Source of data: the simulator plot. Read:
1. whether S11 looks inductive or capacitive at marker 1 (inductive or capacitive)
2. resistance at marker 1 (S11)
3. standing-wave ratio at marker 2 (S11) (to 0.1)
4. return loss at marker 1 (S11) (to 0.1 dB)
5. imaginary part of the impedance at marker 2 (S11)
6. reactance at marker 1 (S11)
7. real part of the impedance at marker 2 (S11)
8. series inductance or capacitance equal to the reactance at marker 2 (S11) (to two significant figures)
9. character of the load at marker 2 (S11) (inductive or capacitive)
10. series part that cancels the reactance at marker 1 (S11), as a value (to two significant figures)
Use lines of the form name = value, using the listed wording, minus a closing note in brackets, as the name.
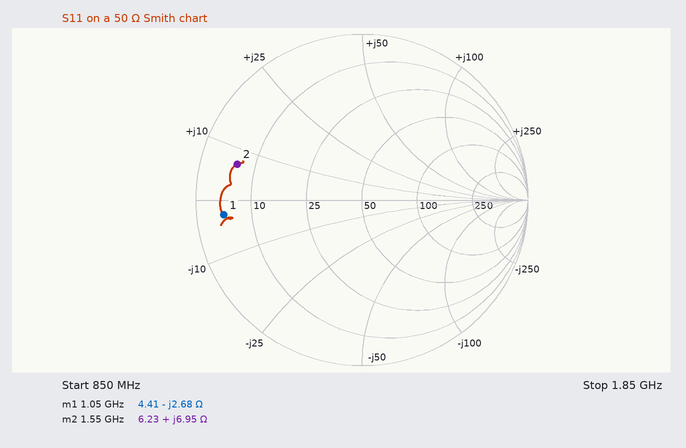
whether S11 looks inductive or capacitive at marker 1 = capacitive
resistance at marker 1 = 4.41 Ω
standing-wave ratio at marker 2 (S11) = 8.2
return loss at marker 1 (S11) = 1.5 dB
imaginary part of the impedance at marker 2 = +6.95 Ω
reactance at marker 1 = -2.68 Ω
real part of the impedance at marker 2 = 6.23 Ω
series inductance or capacitance equal to the reactance at marker 2 (S11) = 710 pH
character of the load at marker 2 (S11) = inductive
series part that cancels the reactance at marker 1 (S11), as a value = 410 pH
